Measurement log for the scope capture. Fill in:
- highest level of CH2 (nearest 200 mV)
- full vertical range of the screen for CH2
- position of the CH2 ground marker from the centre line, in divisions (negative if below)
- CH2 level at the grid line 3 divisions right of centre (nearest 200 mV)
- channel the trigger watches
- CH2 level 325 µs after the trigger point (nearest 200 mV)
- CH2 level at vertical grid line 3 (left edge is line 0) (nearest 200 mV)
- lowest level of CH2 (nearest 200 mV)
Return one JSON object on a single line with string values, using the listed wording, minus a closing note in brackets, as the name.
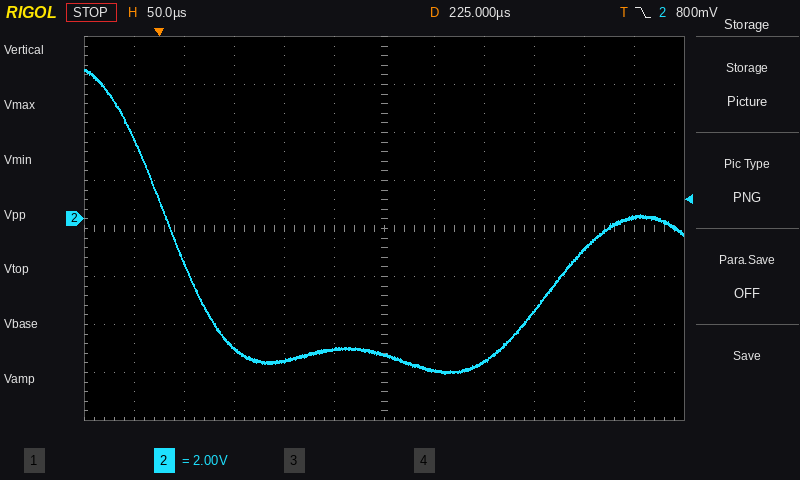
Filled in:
{"highest level of CH2": "6.2 V", "full vertical range of the screen for CH2": "16 V", "position of the CH2 ground marker from the centre line, in divisions": "+0.2 div", "CH2 level at the grid line 3 divisions right of centre": "-3.8 V", "channel the trigger watches": "CH2", "CH2 level 325 µs after the trigger point": "-6.0 V", "CH2 level at vertical grid line 3 (left edge is line 0)": "-5.4 V", "lowest level of CH2": "-6.4 V"}
